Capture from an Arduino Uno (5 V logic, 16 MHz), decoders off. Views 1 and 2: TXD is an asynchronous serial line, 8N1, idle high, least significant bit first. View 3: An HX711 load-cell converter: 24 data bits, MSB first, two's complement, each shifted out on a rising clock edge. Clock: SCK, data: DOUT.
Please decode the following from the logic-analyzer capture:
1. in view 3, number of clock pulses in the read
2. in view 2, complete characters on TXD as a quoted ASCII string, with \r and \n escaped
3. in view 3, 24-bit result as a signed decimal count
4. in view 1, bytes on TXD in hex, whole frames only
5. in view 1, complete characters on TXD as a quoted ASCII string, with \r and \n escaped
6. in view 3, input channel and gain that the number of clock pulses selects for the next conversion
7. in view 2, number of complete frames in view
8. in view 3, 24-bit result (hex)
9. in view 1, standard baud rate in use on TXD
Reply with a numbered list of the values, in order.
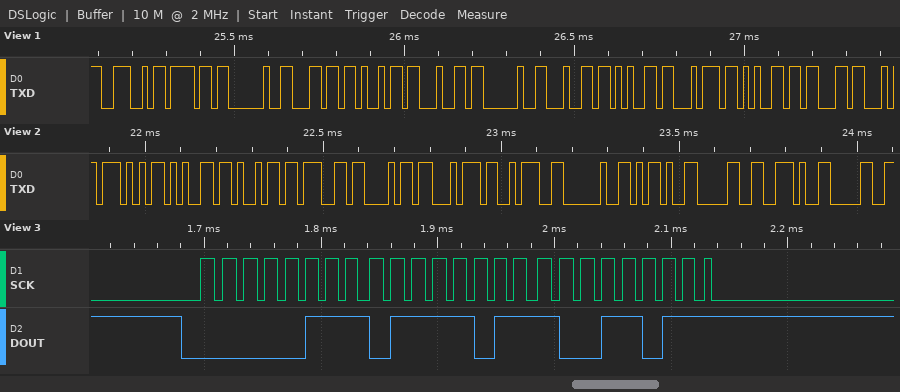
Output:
1. 25
2. "Weight: -0.0"
3. 490395
4. 4E 6F 20 6C 69 64 20 64 65 74 65 63
5. "No lid detec"
6. channel A, gain 128
7. 12
8. 0x077B9B
9. 57600 baud
